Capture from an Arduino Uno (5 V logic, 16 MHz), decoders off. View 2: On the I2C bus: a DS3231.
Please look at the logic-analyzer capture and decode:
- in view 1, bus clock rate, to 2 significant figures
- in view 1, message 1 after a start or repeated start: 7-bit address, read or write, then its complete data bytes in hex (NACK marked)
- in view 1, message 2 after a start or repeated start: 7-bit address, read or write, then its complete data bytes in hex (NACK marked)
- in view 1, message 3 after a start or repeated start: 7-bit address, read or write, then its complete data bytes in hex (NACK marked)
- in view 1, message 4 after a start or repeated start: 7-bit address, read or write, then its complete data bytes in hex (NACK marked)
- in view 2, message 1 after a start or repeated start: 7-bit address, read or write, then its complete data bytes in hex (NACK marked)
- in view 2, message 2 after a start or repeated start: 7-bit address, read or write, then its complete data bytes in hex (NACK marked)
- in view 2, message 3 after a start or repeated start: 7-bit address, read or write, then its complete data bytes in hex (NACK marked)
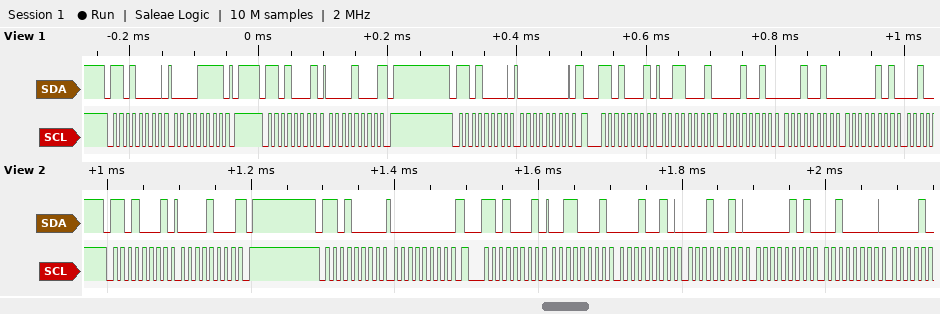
100 kHz
0x68 write: 0F
0x68 read: 08 NACK
0x68 write: 00
0x68 read: 31 12 12 05
0x68 read: 08 NACK
0x68 write: 00
0x68 read: 31 12 12 05 20
